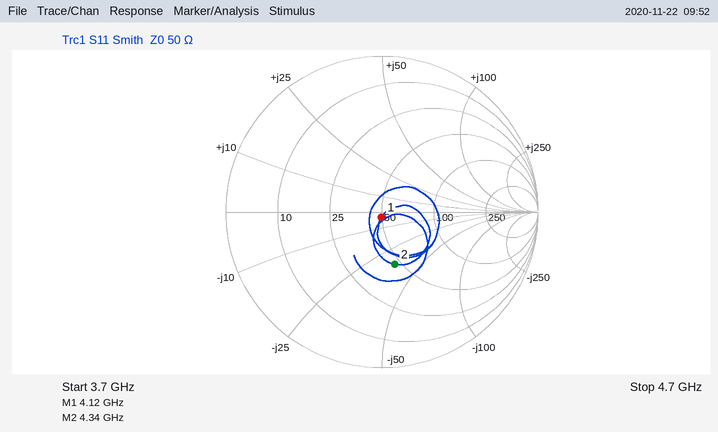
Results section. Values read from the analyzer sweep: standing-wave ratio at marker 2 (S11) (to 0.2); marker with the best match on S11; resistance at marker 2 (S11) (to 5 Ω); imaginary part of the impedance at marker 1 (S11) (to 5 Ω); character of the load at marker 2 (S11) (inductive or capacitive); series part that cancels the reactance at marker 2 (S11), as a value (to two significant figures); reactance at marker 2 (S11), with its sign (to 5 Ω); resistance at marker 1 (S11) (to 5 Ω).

2.0
marker 1
45 Ω
-5 Ω
capacitive
1.3 nH
-35 Ω
50 Ω
